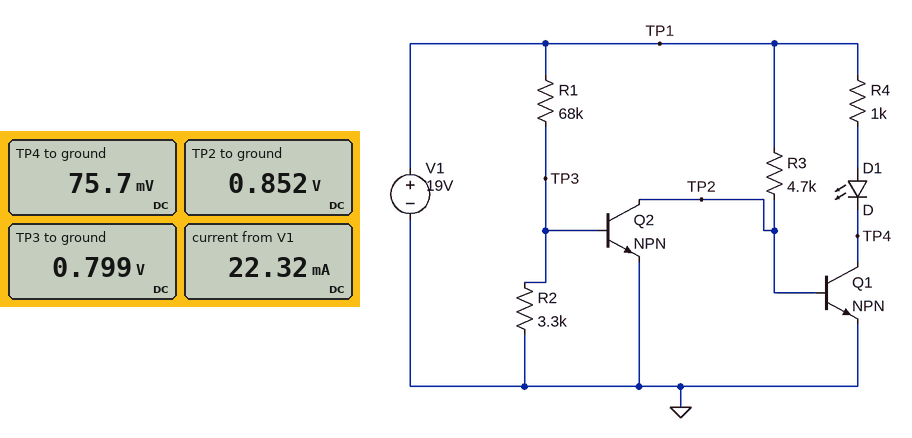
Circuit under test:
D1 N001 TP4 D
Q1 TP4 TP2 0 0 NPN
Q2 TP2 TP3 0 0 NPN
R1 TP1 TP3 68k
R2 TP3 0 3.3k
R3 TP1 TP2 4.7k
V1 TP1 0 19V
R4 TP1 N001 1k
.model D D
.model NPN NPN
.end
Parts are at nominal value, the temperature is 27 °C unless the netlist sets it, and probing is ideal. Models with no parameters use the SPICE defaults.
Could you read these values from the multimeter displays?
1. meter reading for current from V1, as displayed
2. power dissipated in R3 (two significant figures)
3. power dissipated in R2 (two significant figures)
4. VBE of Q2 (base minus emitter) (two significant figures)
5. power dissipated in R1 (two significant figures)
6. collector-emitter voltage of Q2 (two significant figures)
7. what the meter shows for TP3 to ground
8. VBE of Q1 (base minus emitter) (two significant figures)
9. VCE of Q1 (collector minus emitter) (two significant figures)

22.32 mA
70 mW
190 µW
800 mV
4.9 mW
850 mV
0.799 V
850 mV
76 mV
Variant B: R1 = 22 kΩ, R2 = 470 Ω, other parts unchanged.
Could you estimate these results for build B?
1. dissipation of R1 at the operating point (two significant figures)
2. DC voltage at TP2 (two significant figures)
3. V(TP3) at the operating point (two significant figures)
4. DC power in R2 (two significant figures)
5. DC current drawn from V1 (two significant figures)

16 mW
860 mV
400 mV
340 µW
23 mA
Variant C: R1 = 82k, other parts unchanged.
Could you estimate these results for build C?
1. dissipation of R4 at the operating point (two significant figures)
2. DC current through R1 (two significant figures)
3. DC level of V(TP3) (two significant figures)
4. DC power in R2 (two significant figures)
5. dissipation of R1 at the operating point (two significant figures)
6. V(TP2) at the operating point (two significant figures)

330 mW
220 µA
730 mV
160 µW
4.1 mW
860 mV
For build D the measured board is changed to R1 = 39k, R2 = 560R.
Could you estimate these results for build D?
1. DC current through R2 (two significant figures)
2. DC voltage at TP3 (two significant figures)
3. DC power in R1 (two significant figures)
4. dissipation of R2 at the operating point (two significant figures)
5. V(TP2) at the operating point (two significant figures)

480 µA
270 mV
9.0 mW
130 µW
860 mV
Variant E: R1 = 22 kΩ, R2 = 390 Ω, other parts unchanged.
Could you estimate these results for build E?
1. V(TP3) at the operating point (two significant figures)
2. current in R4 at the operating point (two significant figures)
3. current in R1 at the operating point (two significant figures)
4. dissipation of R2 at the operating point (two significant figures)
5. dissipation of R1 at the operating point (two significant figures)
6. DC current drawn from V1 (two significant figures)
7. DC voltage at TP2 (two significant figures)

330 mV
18 mA
850 µA
280 µW
16 mW
23 mA
860 mV
